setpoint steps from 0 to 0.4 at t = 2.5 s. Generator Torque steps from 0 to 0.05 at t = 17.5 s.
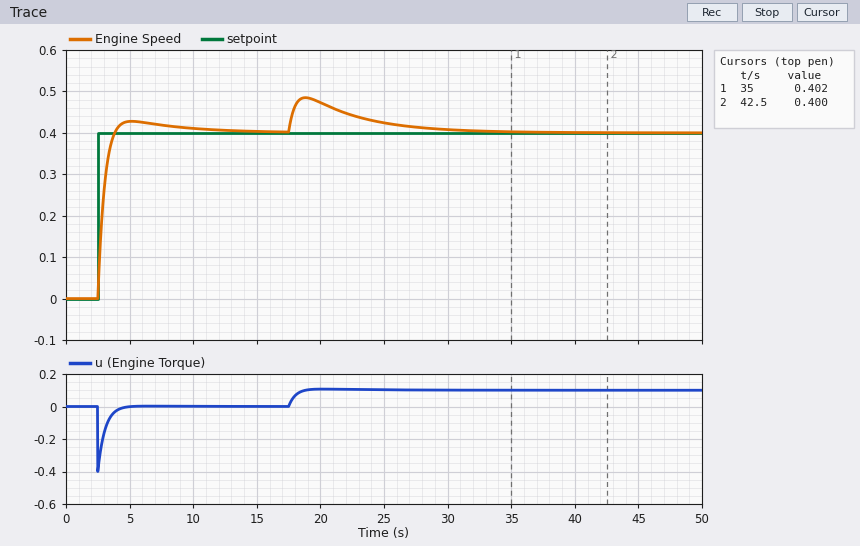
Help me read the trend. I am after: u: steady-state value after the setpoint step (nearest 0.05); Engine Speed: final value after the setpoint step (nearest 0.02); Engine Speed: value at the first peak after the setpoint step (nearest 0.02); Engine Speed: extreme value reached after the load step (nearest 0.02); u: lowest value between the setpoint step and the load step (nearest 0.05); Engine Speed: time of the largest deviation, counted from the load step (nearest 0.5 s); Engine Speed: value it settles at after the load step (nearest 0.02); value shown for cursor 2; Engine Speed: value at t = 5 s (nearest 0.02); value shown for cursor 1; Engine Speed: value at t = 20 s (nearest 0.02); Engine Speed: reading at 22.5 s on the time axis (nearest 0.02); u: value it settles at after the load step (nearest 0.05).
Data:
0.00
0.40
0.42
0.48
-0.40
1.5 s
0.40
0.400
0.42
0.402
0.48
0.44
0.10
